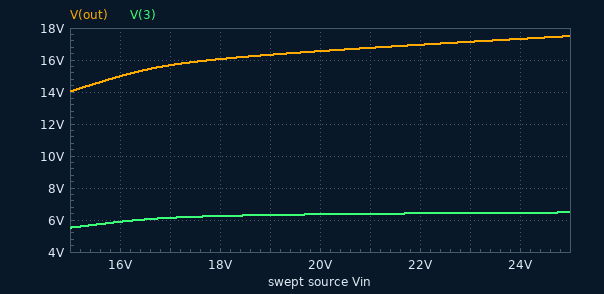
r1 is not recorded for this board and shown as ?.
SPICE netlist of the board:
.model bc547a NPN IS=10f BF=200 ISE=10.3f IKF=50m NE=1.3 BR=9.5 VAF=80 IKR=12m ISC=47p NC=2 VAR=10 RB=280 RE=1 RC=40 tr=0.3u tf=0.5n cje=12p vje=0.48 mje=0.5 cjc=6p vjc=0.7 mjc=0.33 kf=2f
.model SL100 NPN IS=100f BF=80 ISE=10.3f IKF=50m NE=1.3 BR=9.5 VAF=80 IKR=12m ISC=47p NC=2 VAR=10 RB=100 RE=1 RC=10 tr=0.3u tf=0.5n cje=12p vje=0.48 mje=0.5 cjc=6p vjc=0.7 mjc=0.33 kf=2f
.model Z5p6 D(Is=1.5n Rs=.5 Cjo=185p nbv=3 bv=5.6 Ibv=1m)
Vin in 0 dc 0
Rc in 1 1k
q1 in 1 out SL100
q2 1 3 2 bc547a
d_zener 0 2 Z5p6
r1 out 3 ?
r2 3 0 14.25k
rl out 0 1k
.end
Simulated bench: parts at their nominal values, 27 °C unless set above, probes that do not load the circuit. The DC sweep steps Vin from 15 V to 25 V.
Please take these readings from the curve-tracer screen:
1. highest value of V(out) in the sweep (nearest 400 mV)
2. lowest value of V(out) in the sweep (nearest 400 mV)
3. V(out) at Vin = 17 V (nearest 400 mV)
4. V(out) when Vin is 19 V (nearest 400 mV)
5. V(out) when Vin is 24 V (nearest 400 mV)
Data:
17.6 V
14.0 V
15.6 V
16.4 V
17.2 V
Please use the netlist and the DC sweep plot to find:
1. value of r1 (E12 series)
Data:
22 kΩ
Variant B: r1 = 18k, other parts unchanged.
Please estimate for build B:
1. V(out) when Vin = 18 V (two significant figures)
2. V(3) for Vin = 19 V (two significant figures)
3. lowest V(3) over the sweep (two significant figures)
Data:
15 V
6.4 V
6.1 V
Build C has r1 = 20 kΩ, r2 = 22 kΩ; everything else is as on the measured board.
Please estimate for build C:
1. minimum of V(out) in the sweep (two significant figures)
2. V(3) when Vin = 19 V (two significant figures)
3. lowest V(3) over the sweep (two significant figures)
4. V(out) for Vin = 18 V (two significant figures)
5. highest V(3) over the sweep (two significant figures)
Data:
12 V
6.4 V
6.3 V
13 V
6.5 V
